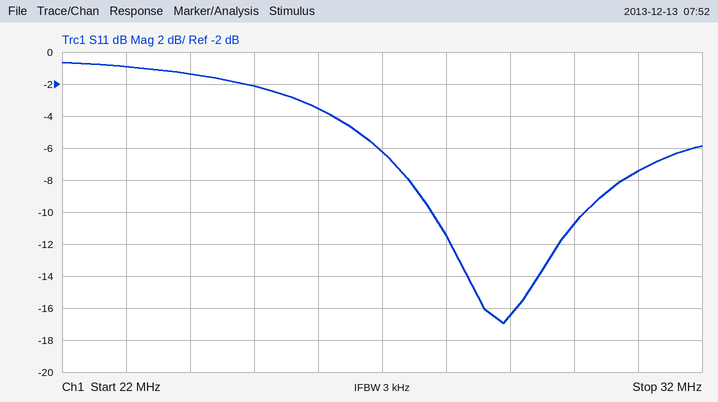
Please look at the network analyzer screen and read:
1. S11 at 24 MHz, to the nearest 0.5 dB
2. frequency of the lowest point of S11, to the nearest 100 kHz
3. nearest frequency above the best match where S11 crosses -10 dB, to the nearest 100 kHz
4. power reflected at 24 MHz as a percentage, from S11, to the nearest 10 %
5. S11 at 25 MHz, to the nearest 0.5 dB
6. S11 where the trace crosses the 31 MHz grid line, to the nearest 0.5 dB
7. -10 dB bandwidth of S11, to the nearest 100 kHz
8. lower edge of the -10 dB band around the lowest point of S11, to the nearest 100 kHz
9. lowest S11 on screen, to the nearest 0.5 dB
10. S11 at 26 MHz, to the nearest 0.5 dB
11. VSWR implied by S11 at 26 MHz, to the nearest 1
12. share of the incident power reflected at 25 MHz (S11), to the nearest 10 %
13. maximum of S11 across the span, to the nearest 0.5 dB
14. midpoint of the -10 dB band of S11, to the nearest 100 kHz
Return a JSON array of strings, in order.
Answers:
["-1.5 dB", "28.9 MHz", "30.2 MHz", "70 %", "-2.0 dB", "-7.5 dB", "2.4 MHz", "27.8 MHz", "-17.0 dB", "-3.5 dB", "5", "60 %", "-0.5 dB", "29.0 MHz"]
